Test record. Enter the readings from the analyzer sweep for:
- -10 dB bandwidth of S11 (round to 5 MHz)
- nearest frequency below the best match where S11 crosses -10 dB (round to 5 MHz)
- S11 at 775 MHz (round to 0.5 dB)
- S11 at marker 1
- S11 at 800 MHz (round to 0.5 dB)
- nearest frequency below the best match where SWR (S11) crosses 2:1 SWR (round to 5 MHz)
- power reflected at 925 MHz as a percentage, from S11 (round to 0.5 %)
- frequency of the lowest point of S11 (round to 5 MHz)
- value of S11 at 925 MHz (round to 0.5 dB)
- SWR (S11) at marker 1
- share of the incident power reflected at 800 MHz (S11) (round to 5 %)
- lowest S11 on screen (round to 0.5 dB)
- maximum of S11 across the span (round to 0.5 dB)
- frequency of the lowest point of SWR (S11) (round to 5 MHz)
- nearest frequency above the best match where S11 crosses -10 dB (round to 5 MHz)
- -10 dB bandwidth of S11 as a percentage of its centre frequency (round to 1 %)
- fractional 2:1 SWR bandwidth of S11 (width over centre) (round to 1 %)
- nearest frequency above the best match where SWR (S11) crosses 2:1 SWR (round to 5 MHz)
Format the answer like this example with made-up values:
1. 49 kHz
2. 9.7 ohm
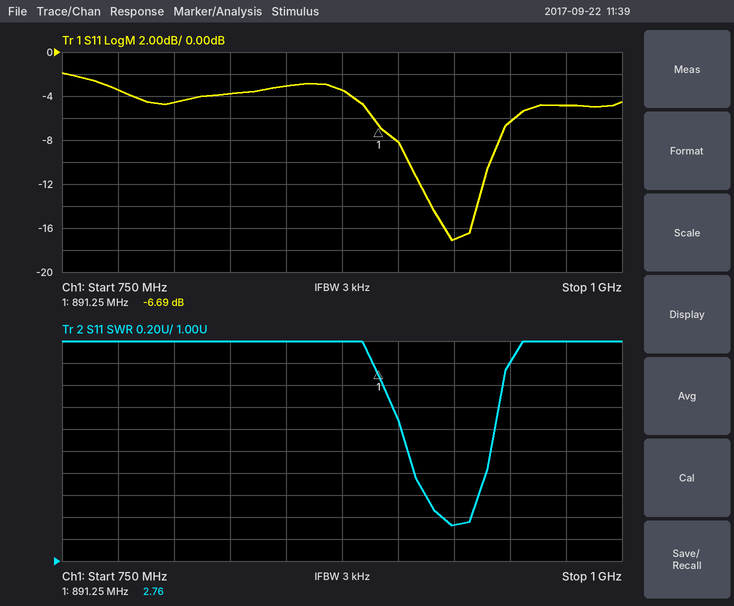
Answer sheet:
1. 35 MHz
2. 905 MHz
3. -3.5 dB
4. -6.69 dB
5. -4.5 dB
6. 905 MHz
7. 2.0 %
8. 925 MHz
9. -17.0 dB
10. 2.76
11. 35 %
12. -17.0 dB
13. -2.0 dB
14. 925 MHz
15. 940 MHz
16. 4 %
17. 4 %
18. 940 MHz
